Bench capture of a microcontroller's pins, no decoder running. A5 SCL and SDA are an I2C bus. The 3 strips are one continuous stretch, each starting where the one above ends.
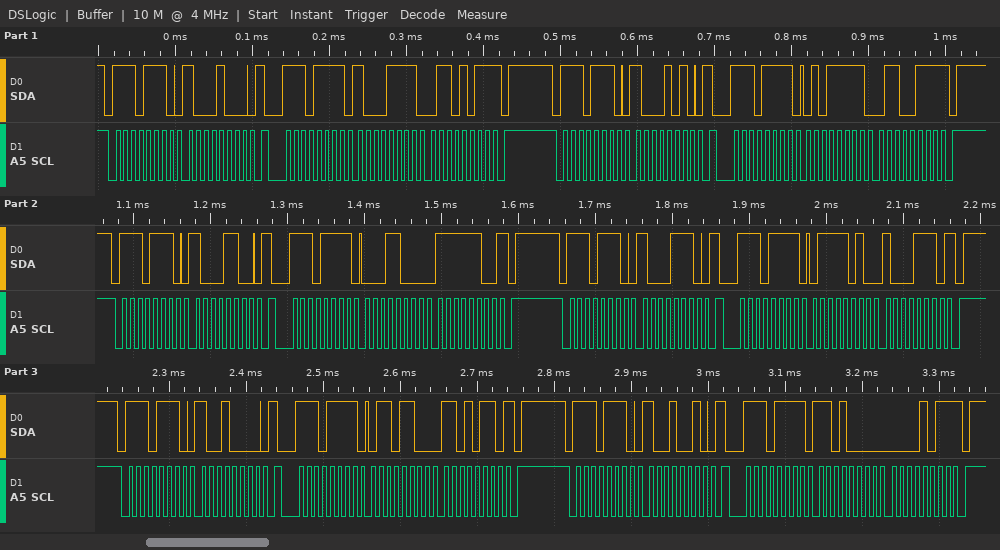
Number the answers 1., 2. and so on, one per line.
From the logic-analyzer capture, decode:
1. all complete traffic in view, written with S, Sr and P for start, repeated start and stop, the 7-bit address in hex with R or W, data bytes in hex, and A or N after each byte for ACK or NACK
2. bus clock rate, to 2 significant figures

1. S 77W A 88 A Sr 77R A 8F A 6B N P S 77W A 8A A Sr 77R A 5F A 67 N P S 77W A 8C A Sr 77R A 18 A FC N P S 77W A 8E A Sr 77R A 7A A 8E N P S 77W A 90 A Sr 77R A 6C A D6 N P S 77W A 92 A Sr 77R A D0 A 0B N P
2. 100 kHz
